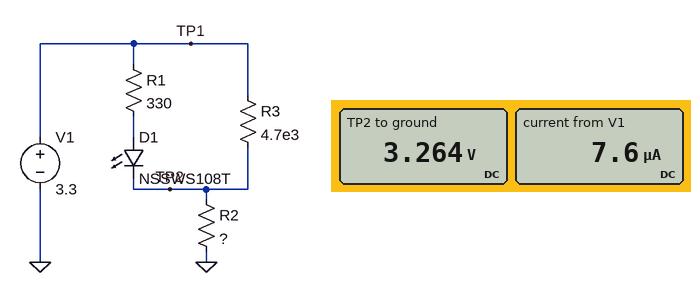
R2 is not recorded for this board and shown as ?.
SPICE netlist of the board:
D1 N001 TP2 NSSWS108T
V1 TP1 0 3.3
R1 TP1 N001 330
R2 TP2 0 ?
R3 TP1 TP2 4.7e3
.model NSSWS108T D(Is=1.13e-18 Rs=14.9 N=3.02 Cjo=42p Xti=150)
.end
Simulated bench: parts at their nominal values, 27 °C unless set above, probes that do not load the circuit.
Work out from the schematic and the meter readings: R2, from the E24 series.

430 kΩ
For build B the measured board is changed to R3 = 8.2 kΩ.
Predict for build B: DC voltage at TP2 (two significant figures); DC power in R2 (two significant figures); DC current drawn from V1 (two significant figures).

3.2 V
24 µW
7.5 µA
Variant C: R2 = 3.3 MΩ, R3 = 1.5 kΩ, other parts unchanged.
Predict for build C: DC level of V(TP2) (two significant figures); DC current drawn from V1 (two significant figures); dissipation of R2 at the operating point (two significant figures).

3.3 V
1.0 µA
3.3 µW
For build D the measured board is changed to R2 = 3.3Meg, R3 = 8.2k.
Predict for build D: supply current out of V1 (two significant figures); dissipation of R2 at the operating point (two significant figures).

1.0 µA
3.3 µW
